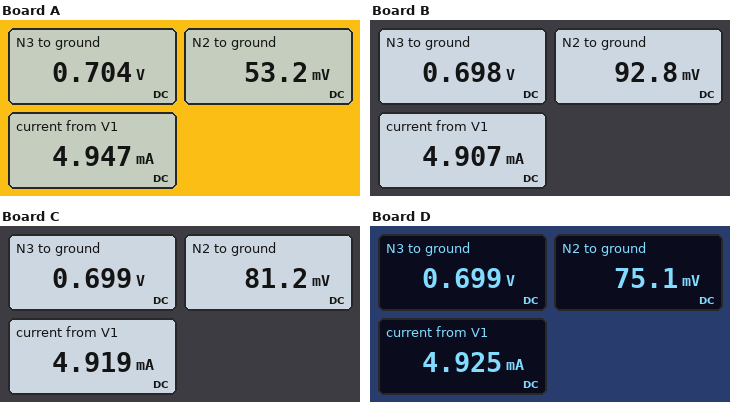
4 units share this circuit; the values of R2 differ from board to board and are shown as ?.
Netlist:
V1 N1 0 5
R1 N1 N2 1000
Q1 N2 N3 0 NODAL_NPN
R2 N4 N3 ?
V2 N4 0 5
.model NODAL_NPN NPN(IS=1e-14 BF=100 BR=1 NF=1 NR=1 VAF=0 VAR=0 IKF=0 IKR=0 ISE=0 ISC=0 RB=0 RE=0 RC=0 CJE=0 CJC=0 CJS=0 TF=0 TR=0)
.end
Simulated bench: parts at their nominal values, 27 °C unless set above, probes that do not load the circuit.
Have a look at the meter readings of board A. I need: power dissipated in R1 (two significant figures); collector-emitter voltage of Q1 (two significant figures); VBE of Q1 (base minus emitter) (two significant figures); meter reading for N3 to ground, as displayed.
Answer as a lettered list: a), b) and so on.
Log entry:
a) 24 mW
b) 53 mV
c) 700 mV
d) 0.704 V
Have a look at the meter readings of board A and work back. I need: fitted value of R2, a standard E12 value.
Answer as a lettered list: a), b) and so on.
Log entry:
a) 4.7 kΩ
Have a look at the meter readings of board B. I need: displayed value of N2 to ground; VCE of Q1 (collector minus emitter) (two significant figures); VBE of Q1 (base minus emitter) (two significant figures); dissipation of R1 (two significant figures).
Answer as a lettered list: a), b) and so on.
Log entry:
a) 92.8 mV
b) 93 mV
c) 700 mV
d) 24 mW
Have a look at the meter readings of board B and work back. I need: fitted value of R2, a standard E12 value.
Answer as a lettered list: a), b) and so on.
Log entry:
a) 22 kΩ
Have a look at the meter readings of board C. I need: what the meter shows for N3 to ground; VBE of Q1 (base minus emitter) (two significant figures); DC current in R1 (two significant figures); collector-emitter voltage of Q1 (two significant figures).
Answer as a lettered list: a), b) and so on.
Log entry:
a) 0.699 V
b) 700 mV
c) 4.9 mA
d) 81 mV
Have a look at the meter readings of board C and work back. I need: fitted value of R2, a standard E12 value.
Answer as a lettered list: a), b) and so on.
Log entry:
a) 15 kΩ
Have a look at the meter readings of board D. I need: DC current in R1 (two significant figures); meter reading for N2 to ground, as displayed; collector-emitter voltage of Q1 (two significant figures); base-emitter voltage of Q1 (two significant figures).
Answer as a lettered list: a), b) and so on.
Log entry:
a) 4.9 mA
b) 75.1 mV
c) 75 mV
d) 700 mV
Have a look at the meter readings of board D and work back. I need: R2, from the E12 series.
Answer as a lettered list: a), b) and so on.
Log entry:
a) 12 kΩ
